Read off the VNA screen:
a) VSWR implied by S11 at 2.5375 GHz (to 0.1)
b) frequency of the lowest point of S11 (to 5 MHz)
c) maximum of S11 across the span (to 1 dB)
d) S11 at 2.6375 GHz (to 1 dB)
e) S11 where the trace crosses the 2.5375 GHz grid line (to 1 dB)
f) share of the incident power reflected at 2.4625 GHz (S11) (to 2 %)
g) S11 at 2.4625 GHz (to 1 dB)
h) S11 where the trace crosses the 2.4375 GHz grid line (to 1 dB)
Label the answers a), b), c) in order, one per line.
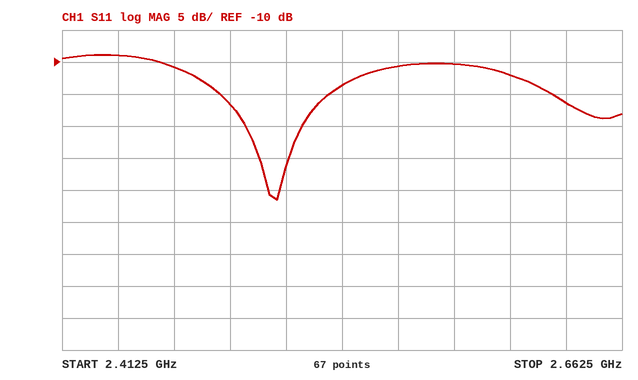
a) 1.5
b) 2.510 GHz
c) -9 dB
d) -16 dB
e) -14 dB
f) 8 %
g) -11 dB
h) -9 dB
